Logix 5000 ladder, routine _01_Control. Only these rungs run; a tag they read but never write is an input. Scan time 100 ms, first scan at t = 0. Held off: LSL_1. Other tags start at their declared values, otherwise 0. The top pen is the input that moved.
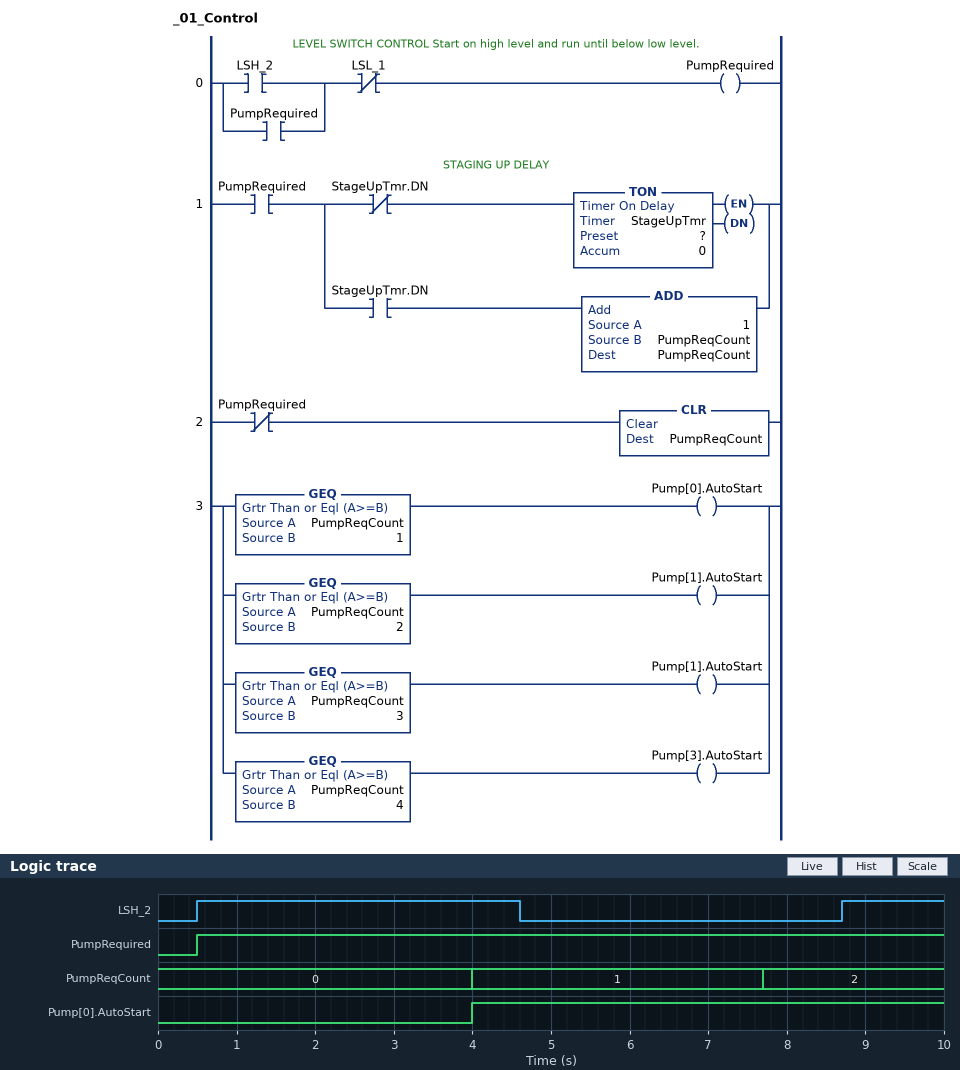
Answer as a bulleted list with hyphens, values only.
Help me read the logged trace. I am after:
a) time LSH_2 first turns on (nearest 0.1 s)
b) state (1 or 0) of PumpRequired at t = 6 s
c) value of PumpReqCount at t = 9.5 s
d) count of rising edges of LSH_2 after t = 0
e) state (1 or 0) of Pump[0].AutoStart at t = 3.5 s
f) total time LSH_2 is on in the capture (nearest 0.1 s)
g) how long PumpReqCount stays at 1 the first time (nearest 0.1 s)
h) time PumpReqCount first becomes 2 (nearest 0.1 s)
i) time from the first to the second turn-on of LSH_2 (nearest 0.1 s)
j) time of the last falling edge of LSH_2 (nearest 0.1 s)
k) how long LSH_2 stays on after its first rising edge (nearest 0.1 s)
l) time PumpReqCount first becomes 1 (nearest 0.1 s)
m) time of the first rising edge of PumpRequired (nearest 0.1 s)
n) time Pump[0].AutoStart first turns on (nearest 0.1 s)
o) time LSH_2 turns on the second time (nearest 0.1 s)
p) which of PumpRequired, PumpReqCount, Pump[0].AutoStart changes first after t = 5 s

- 0.5 s
- 1
- 2
- 2
- 0
- 5.4 s
- 3.7 s
- 7.7 s
- 8.2 s
- 4.6 s
- 4.1 s
- 4.0 s
- 0.5 s
- 4.0 s
- 8.7 s
- PumpReqCount
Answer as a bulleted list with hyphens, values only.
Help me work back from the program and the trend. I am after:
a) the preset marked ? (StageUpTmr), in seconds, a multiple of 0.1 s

- 3.5 s
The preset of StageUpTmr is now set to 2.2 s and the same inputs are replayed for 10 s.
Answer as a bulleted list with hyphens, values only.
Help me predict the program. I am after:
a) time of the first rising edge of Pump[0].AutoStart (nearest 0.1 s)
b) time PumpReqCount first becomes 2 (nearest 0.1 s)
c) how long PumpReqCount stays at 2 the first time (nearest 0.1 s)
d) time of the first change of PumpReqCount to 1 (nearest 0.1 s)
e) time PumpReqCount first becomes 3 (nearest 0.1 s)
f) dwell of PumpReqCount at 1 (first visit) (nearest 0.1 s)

- 2.7 s
- 5.1 s
- 2.4 s
- 2.7 s
- 7.5 s
- 2.4 s
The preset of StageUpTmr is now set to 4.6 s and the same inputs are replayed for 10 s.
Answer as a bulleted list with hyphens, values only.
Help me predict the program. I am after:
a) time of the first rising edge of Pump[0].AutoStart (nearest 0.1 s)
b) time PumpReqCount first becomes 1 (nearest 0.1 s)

- 5.1 s
- 5.1 s
